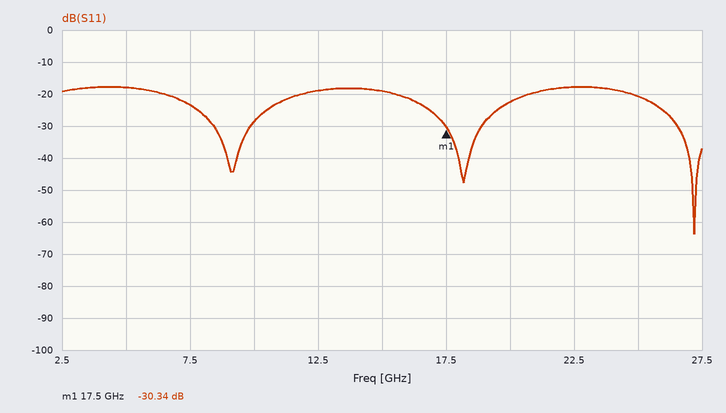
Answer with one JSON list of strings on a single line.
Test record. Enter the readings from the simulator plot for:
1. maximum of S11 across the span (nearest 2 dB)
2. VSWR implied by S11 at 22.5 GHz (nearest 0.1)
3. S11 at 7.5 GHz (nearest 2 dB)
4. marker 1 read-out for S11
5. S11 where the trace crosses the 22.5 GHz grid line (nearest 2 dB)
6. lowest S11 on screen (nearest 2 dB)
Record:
["-18 dB", "1.3", "-24 dB", "-30.34 dB", "-18 dB", "-64 dB"]
